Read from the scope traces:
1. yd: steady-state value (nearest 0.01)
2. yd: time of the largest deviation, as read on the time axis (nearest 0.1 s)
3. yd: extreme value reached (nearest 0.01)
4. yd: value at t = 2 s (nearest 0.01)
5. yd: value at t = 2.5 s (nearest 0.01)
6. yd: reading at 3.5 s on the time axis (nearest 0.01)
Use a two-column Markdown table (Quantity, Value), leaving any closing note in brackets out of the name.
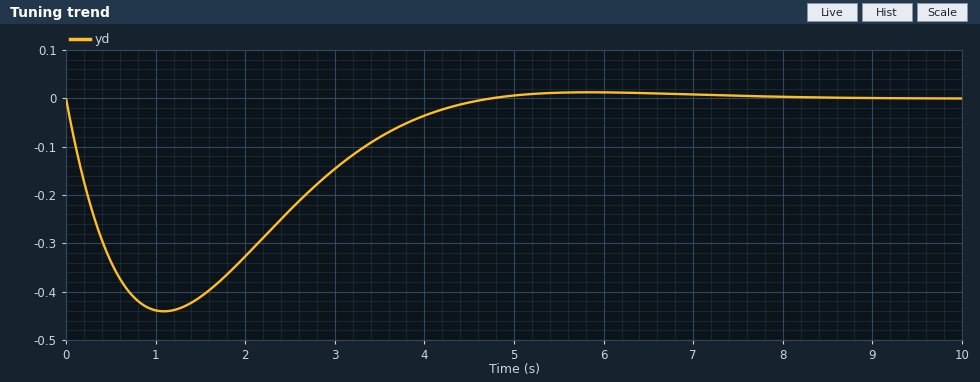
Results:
| Quantity | Value |
|---|---|
| yd: steady-state value | 0.00 |
| yd: time of the largest deviation, as read on the time axis | 1.1 s |
| yd: extreme value reached | -0.44 |
| yd: value at t = 2 s | -0.33 |
| yd: value at t = 2.5 s | -0.23 |
| yd: reading at 3.5 s on the time axis | -0.08 |
